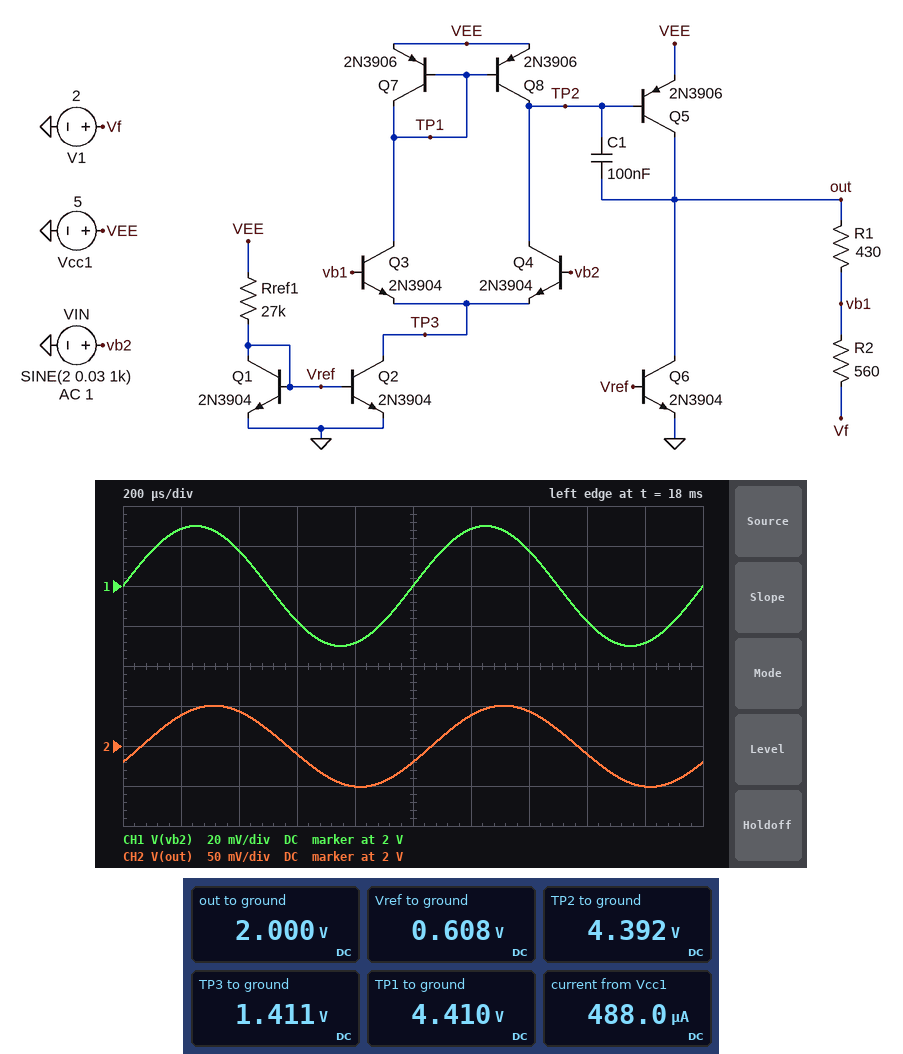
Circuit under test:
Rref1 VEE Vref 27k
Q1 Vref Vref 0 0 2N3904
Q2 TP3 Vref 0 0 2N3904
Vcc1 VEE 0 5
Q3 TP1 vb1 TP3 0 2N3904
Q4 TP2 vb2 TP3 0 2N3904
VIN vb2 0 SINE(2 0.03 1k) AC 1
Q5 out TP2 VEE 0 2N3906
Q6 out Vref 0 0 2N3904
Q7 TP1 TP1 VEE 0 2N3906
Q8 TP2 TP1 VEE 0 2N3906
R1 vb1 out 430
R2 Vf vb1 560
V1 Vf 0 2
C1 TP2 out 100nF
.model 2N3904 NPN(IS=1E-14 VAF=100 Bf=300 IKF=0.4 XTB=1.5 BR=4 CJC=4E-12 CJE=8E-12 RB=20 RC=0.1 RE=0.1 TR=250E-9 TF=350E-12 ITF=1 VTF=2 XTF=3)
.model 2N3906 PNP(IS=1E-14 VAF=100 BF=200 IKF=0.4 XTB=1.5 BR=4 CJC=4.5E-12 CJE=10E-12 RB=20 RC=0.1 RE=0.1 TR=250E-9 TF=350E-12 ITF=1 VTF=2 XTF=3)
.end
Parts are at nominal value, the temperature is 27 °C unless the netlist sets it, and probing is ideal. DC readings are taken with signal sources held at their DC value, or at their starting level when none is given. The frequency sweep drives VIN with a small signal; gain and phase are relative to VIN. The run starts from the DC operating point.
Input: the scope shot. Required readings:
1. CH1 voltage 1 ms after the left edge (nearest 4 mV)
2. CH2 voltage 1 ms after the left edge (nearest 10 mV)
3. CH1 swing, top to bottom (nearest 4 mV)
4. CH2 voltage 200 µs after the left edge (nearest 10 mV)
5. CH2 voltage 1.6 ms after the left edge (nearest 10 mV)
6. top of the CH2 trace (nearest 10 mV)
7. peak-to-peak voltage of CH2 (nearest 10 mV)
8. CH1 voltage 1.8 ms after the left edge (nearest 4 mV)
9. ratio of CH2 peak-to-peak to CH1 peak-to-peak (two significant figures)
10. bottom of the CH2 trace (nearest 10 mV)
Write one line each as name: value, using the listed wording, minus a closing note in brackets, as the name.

CH1 voltage 1 ms after the left edge: 2.000 V
CH2 voltage 1 ms after the left edge: 1.98 V
CH1 swing, top to bottom: 60 mV
CH2 voltage 200 µs after the left edge: 2.04 V
CH2 voltage 1.6 ms after the left edge: 1.99 V
top of the CH2 trace: 2.05 V
peak-to-peak voltage of CH2: 100 mV
CH1 voltage 1.8 ms after the left edge: 1.972 V
ratio of CH2 peak-to-peak to CH1 peak-to-peak: 1.7
bottom of the CH2 trace: 1.95 V
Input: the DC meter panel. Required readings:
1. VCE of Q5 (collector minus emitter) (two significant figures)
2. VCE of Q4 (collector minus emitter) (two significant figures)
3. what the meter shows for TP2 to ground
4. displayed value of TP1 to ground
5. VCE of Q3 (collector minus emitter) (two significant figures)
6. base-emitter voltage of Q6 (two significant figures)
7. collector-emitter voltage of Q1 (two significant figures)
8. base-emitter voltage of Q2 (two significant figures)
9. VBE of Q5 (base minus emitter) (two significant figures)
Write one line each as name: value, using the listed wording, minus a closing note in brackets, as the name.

VCE of Q5 (collector minus emitter): -3.0 V
VCE of Q4 (collector minus emitter): 3.0 V
what the meter shows for TP2 to ground: 4.392 V
displayed value of TP1 to ground: 4.410 V
VCE of Q3 (collector minus emitter): 3.0 V
base-emitter voltage of Q6: 610 mV
collector-emitter voltage of Q1: 610 mV
base-emitter voltage of Q2: 610 mV
VBE of Q5 (base minus emitter): -610 mV
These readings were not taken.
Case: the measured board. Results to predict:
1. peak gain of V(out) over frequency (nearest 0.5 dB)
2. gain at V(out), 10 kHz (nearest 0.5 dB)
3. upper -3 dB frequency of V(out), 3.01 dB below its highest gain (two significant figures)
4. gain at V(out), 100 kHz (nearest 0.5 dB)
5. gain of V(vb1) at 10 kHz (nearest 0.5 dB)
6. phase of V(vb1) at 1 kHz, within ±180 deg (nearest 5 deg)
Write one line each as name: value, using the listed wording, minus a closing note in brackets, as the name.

peak gain of V(out) over frequency: 5.0 dB
gain at V(out), 10 kHz: -2.5 dB
upper -3 dB frequency of V(out), 3.01 dB below its highest gain: 3.5 kHz
gain at V(out), 100 kHz: -5.0 dB
gain of V(vb1) at 10 kHz: -7.5 dB
phase of V(vb1) at 1 kHz, within ±180 deg: -25 deg
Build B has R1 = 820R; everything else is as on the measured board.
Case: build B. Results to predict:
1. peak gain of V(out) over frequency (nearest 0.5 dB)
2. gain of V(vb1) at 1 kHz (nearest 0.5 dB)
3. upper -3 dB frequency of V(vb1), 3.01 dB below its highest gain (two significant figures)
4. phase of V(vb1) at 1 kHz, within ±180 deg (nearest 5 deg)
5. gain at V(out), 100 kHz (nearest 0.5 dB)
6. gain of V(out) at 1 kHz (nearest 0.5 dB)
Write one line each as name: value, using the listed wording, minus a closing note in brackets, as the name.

peak gain of V(out) over frequency: 8.0 dB
gain of V(vb1) at 1 kHz: -1.0 dB
upper -3 dB frequency of V(vb1), 3.01 dB below its highest gain: 2.3 kHz
phase of V(vb1) at 1 kHz, within ±180 deg: -30 deg
gain at V(out), 100 kHz: -5.5 dB
gain of V(out) at 1 kHz: 7.0 dB
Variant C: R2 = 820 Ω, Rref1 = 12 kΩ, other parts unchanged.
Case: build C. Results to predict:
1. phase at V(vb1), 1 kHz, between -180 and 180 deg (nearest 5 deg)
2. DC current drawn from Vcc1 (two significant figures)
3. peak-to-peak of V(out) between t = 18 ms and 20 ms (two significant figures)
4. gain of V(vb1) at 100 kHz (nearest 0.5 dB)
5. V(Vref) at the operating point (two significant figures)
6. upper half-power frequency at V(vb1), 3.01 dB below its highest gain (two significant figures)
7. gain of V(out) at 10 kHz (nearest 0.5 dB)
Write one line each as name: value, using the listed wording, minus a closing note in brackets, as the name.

phase at V(vb1), 1 kHz, between -180 and 180 deg: -10 deg
DC current drawn from Vcc1: 1.1 mA
peak-to-peak of V(out) between t = 18 ms and 20 ms: 91 mV
gain of V(vb1) at 100 kHz: -7.0 dB
V(Vref) at the operating point: 630 mV
upper half-power frequency at V(vb1), 3.01 dB below its highest gain: 12 kHz
gain of V(out) at 10 kHz: 1.5 dB
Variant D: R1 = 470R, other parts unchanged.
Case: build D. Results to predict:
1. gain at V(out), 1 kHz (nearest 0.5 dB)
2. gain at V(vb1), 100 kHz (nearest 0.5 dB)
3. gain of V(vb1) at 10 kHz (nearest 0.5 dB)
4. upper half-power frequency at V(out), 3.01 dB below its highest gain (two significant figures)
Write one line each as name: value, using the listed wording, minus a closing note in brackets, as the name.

gain at V(out), 1 kHz: 5.0 dB
gain at V(vb1), 100 kHz: -10.5 dB
gain of V(vb1) at 10 kHz: -8.0 dB
upper half-power frequency at V(out), 3.01 dB below its highest gain: 3.3 kHz
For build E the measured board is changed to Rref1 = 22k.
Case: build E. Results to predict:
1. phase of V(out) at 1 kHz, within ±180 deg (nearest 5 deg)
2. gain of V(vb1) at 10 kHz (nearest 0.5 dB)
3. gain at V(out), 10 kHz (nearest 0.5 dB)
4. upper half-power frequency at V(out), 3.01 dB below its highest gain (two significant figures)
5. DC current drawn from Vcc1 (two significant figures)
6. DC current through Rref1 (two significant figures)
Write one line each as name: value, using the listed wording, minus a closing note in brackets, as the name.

phase of V(out) at 1 kHz, within ±180 deg: -20 deg
gain of V(vb1) at 10 kHz: -6.5 dB
gain at V(out), 10 kHz: -1.5 dB
upper half-power frequency at V(out), 3.01 dB below its highest gain: 4.5 kHz
DC current drawn from Vcc1: 600 µA
DC current through Rref1: 200 µA
